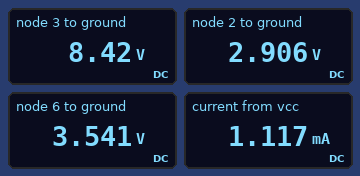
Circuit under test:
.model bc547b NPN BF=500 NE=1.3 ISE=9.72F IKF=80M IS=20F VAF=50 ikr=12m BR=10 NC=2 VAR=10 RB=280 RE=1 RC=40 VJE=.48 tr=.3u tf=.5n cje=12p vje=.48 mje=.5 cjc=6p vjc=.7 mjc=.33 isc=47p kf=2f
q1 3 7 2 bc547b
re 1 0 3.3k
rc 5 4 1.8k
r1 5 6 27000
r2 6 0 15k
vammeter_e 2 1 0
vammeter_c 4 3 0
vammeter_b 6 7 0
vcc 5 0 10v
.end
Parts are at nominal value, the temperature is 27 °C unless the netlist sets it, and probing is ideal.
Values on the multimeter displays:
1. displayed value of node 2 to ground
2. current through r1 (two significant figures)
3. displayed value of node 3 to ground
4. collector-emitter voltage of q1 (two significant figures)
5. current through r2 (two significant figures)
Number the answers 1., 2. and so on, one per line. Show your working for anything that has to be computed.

1. 2.906 V
2. (10 V - 3.541 V) / 27 kΩ = 240 µA
3. 8.42 V
4. 8.42 V - 2.906 V = 5.5 V
5. (3.541 V) / 15 kΩ = 240 µA
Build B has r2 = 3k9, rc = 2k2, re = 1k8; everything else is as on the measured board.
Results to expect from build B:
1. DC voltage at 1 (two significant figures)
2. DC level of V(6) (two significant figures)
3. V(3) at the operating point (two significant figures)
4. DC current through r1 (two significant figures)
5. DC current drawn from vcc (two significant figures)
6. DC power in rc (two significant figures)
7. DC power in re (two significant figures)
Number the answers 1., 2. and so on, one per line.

1. 650 mV
2. 1.3 V
3. 9.2 V
4. 320 µA
5. 680 µA
6. 280 µW
7. 230 µW
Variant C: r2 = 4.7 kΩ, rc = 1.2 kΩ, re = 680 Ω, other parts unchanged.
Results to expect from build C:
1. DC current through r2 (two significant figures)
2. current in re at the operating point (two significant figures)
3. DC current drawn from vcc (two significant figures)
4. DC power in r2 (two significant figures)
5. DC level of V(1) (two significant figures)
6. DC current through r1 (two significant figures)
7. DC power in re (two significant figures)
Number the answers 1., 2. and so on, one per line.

1. 310 µA
2. 1.2 mA
3. 1.5 mA
4. 460 µW
5. 820 mV
6. 320 µA
7. 1.0 mW
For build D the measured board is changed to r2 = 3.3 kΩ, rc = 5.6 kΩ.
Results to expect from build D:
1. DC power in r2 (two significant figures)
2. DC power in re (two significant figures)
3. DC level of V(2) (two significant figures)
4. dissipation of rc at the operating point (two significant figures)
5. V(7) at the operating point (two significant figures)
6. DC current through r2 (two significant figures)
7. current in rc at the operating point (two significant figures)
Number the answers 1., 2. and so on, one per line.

1. 360 µW
2. 76 µW
3. 500 mV
4. 130 µW
5. 1.1 V
6. 330 µA
7. 150 µA
